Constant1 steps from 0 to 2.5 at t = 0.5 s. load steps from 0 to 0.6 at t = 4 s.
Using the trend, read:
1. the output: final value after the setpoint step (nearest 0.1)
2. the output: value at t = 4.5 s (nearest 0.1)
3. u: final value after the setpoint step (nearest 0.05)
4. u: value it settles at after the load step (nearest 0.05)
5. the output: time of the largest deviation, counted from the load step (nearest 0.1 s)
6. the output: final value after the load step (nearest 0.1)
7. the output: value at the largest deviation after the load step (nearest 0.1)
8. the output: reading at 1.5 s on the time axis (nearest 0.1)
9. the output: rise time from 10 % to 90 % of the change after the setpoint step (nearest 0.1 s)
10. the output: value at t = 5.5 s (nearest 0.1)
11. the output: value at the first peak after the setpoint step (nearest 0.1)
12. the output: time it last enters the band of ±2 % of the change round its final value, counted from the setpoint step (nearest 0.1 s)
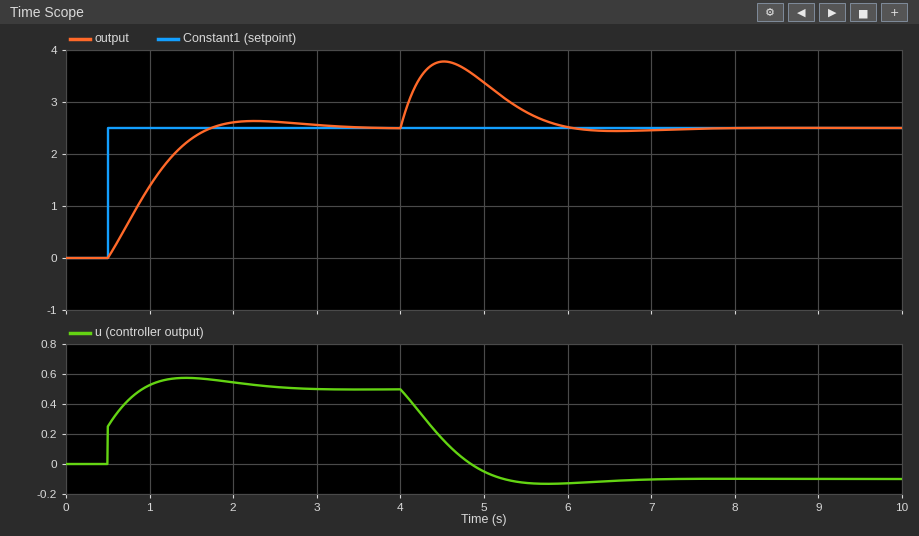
2.5
3.8
0.50
-0.10
0.5 s
2.5
3.8
2.3
0.9 s
2.8
2.6
2.6 s
